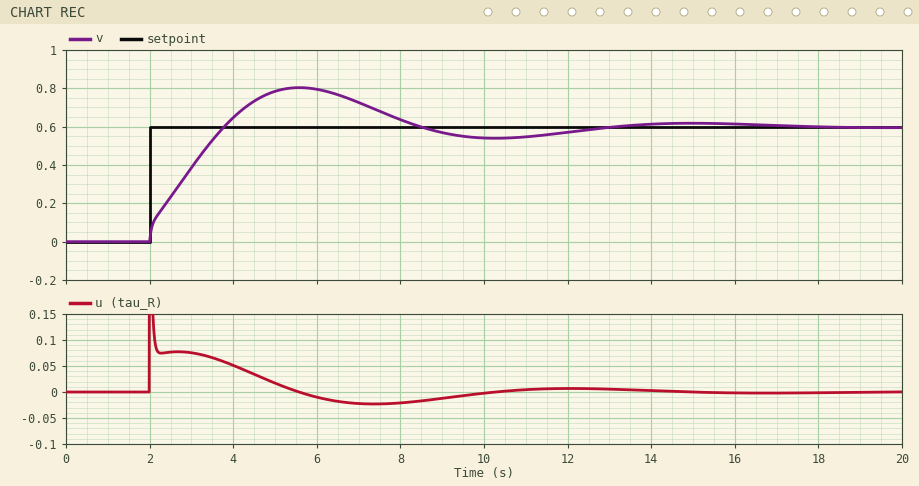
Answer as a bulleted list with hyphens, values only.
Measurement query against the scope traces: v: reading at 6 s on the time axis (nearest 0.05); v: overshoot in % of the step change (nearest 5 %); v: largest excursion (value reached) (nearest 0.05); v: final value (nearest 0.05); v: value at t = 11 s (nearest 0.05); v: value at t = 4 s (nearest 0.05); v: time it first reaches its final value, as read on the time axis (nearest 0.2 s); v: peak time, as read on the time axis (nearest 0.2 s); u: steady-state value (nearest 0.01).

- 0.80
- 35 %
- 0.80
- 0.60
- 0.55
- 0.65
- 3.8 s
- 5.6 s
- 0.00
